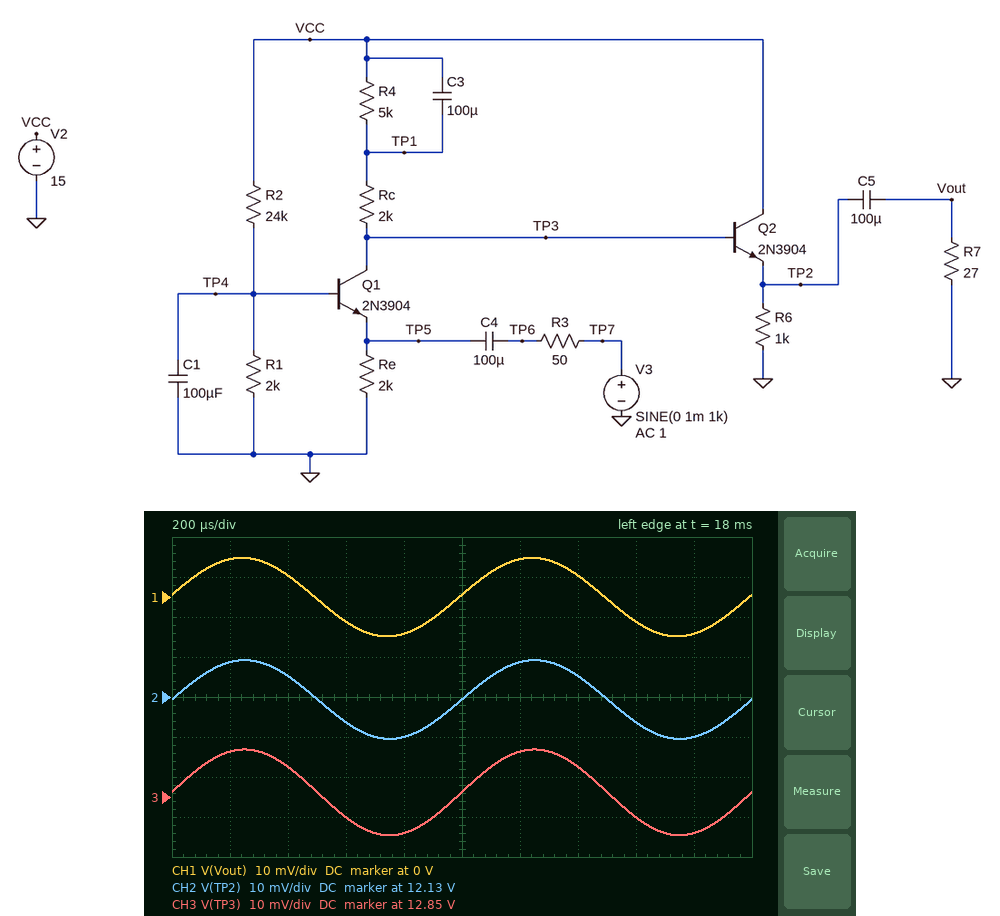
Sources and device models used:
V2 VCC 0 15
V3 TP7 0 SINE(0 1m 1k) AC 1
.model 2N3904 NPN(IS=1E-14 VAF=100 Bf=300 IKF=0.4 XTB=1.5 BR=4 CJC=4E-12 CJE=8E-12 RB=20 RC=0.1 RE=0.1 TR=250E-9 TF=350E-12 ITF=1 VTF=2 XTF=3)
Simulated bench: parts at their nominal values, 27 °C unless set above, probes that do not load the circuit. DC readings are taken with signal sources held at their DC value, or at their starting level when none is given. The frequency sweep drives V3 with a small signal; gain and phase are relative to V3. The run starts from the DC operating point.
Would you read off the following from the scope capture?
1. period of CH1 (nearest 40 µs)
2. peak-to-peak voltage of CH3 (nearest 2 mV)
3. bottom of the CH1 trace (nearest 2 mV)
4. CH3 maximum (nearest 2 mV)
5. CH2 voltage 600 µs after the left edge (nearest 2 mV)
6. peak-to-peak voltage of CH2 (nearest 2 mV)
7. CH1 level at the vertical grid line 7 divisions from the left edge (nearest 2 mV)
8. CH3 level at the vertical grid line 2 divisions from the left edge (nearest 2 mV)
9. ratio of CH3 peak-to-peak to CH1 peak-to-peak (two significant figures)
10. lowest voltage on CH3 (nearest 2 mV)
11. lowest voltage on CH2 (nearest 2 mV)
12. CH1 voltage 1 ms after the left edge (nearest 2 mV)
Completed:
1.00 ms
22 mV
-10 mV
12.862 V
12.124 V
20 mV
6 mV
12.858 V
1.1
12.840 V
12.120 V
0 V
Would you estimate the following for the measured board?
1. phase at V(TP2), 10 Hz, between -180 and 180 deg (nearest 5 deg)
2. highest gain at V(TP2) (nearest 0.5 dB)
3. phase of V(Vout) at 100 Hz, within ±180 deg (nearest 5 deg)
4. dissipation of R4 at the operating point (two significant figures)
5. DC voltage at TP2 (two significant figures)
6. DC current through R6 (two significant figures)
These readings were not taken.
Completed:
40 deg
21.0 dB
30 deg
470 µW
12 V
12 mA
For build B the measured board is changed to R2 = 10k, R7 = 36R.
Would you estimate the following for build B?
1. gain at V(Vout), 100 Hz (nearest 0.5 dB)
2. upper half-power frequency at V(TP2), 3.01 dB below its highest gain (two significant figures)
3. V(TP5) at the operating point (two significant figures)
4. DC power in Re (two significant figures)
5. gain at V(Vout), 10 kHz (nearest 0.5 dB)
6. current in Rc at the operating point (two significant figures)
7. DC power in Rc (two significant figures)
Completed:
25.0 dB
6.1 MHz
1.8 V
1.7 mW
26.0 dB
940 µA
1.8 mW
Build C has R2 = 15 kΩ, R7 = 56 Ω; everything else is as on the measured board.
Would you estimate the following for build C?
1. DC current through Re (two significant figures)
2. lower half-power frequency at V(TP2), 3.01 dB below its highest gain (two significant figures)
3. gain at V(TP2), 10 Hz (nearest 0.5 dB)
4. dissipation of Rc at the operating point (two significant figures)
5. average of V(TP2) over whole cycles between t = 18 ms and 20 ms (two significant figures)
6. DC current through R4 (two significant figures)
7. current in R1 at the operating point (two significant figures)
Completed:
560 µA
13 Hz
20.0 dB
700 µW
10 V
590 µA
880 µA
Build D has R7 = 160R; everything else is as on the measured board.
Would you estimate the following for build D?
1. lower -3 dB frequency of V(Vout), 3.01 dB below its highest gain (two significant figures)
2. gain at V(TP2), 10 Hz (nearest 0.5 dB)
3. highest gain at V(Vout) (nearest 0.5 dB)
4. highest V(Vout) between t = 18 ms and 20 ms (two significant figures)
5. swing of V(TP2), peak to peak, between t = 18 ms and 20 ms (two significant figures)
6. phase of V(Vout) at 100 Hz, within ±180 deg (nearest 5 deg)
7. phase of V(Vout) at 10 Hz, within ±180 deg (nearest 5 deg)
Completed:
16 Hz
18.5 dB
22.0 dB
12 mV
25 mV
10 deg
85 deg
